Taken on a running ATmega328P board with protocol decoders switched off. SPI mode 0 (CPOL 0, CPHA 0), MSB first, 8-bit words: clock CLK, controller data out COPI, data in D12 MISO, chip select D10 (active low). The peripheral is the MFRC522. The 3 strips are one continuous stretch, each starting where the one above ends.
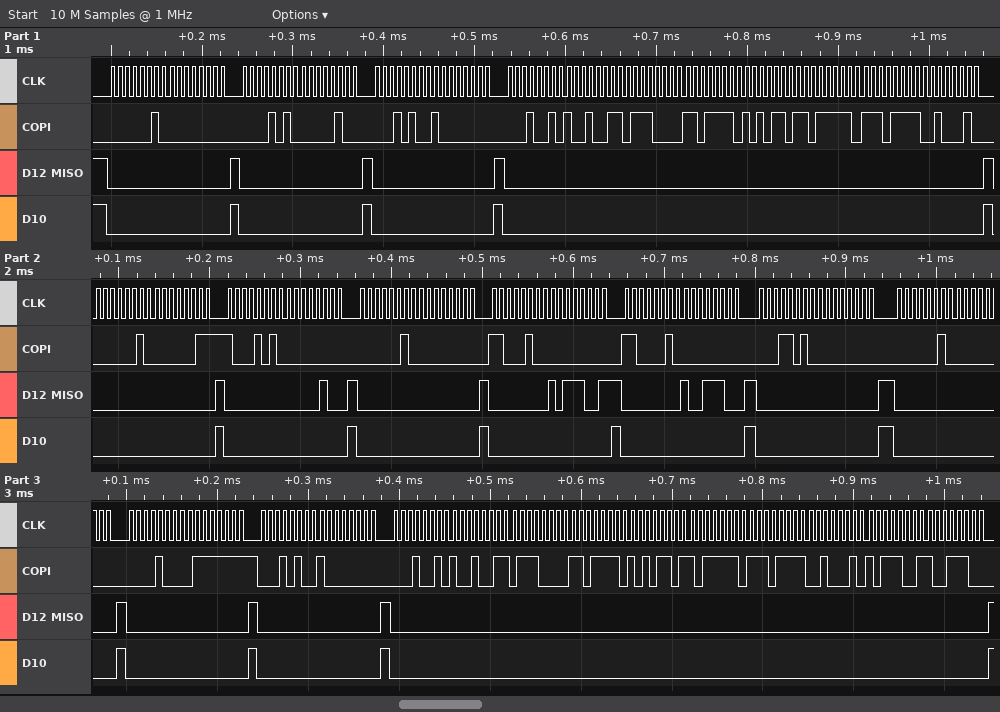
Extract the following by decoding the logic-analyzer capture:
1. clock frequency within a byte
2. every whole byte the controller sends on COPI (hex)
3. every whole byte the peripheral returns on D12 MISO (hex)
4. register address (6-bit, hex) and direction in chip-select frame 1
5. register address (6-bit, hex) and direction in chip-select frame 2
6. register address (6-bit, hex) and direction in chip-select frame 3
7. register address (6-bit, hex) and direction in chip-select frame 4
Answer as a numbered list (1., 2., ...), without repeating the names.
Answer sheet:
1. 125 kHz
2. 02 00 0A 04 14 80 12 93 70 DE AD BE EF 22 02 03 8A 00 02 00 C4 00 C2 00 1A 00 02 00 08 7F 14 80 12 93 70 DE AD BE EF 22 B9 9C
3. 00 00 00 00 00 00 00 00 00 00 00 00 00 00 00 00 00 04 00 00 00 B9 00 9C 00 00 00 00 00 00 00 00 00 00 00 00 00 00 00 00 00 00
4. 0x01 write
5. 0x05 write
6. 0x0A write
7. 0x09 write
